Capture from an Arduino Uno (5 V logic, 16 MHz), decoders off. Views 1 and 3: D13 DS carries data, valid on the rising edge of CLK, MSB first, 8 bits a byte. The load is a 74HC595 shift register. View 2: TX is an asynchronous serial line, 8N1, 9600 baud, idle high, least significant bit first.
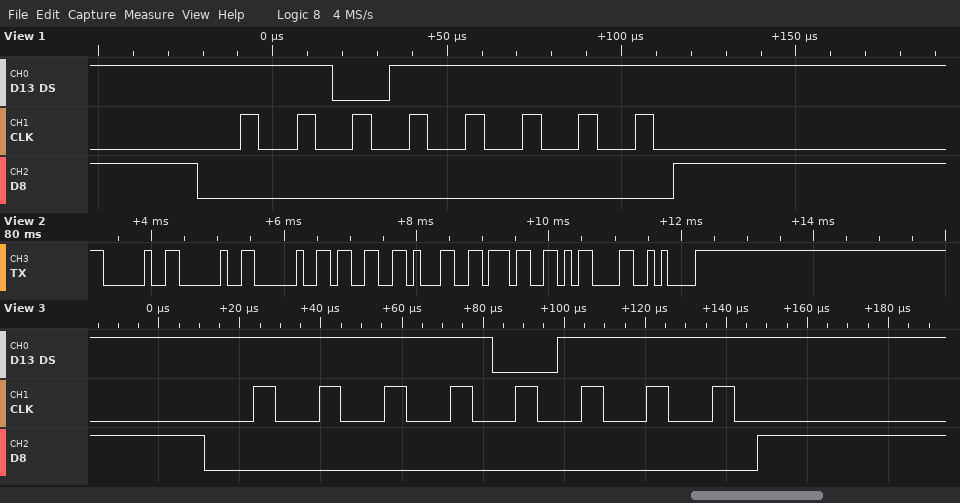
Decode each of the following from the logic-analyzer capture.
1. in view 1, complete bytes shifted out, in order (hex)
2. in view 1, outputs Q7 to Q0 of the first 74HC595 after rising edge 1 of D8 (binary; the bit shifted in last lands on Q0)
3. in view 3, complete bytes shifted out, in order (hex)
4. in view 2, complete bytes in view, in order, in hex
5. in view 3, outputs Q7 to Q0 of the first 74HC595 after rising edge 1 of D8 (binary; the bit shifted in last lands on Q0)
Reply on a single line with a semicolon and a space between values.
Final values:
DF; 11011111; F7; 20 20 20 33 31 37 0D 0A; 11110111
